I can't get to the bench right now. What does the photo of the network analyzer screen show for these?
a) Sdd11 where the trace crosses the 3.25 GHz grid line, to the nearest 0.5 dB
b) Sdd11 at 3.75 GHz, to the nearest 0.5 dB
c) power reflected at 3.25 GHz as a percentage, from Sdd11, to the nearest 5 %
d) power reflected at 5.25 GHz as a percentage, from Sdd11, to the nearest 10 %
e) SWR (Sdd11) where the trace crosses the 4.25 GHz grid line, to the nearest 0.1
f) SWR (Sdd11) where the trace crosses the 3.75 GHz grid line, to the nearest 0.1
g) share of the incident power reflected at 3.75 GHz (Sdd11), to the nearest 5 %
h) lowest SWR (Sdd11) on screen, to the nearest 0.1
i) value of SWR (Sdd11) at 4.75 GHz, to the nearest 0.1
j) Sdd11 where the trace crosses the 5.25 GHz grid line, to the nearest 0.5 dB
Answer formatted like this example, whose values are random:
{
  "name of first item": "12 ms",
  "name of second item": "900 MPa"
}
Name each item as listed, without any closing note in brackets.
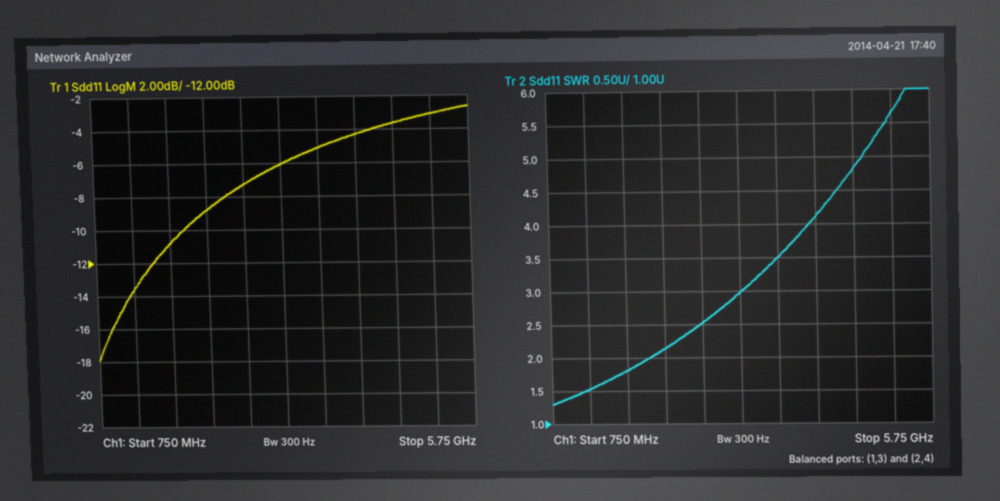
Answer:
{
  "Sdd11 where the trace crosses the 3.25 GHz grid line, to the nearest 0.5 dB": "-6.0 dB",
  "Sdd11 at 3.75 GHz, to the nearest 0.5 dB": "-5.0 dB",
  "power reflected at 3.25 GHz as a percentage, from Sdd11, to the nearest 5 %": "25 %",
  "power reflected at 5.25 GHz as a percentage, from Sdd11, to the nearest 10 %": "50 %",
  "SWR (Sdd11) where the trace crosses the 4.25 GHz grid line, to the nearest 0.1": "4.1",
  "SWR (Sdd11) where the trace crosses the 3.75 GHz grid line, to the nearest 0.1": "3.5",
  "share of the incident power reflected at 3.75 GHz (Sdd11), to the nearest 5 %": "30 %",
  "lowest SWR (Sdd11) on screen, to the nearest 0.1": "1.3",
  "value of SWR (Sdd11) at 4.75 GHz, to the nearest 0.1": "4.8",
  "Sdd11 where the trace crosses the 5.25 GHz grid line, to the nearest 0.5 dB": "-3.0 dB"
}
